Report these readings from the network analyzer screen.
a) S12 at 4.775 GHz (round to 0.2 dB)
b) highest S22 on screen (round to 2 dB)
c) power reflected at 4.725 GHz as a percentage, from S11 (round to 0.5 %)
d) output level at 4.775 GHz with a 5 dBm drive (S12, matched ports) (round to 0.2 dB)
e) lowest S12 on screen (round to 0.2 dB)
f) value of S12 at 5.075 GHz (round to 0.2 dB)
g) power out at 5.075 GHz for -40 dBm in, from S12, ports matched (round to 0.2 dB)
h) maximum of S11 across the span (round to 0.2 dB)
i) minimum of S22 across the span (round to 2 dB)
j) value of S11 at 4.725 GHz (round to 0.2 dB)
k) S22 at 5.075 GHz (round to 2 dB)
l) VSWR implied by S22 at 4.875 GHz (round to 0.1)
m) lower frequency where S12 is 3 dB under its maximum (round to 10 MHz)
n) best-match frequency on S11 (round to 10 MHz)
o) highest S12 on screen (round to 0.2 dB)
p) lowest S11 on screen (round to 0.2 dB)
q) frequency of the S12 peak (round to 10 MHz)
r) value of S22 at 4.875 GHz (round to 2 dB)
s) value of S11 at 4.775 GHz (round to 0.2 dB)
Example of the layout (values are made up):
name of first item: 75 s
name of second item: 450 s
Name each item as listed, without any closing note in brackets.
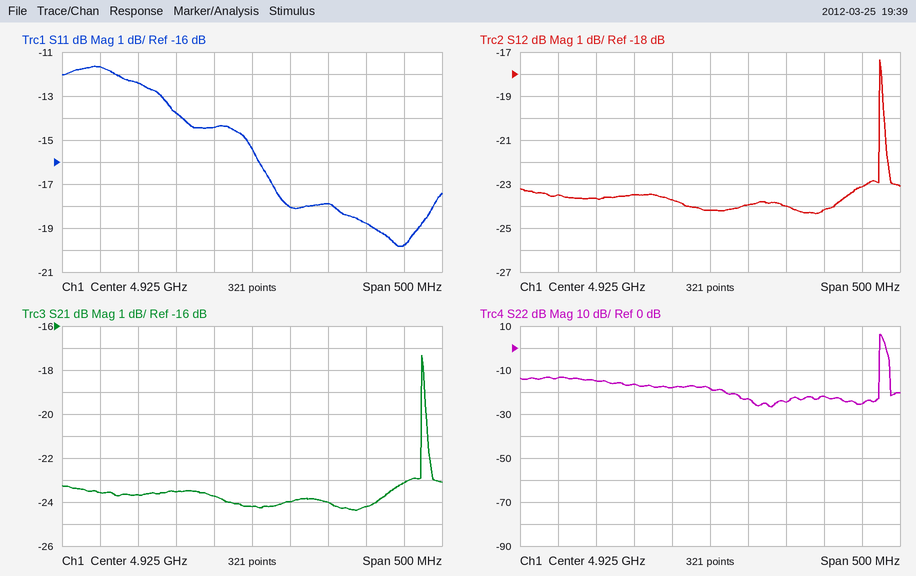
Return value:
S12 at 4.775 GHz: -23.6 dB
highest S22 on screen: 6 dB
power reflected at 4.725 GHz as a percentage, from S11: 7.0 %
output level at 4.775 GHz with a 5 dBm drive (S12, matched ports): -18.6 dBm
lowest S12 on screen: -24.4 dB
value of S12 at 5.075 GHz: -24.2 dB
power out at 5.075 GHz for -40 dBm in, from S12, ports matched: -64.2 dBm
maximum of S11 across the span: -11.6 dB
minimum of S22 across the span: -26 dB
value of S11 at 4.725 GHz: -11.6 dB
S22 at 5.075 GHz: -22 dB
VSWR implied by S22 at 4.875 GHz: 1.3
lower frequency where S12 is 3 dB under its maximum: 5.15 GHz
best-match frequency on S11: 5.12 GHz
highest S12 on screen: -17.4 dB
lowest S11 on screen: -19.8 dB
frequency of the S12 peak: 5.15 GHz
value of S22 at 4.875 GHz: -18 dB
value of S11 at 4.775 GHz: -12.4 dB
